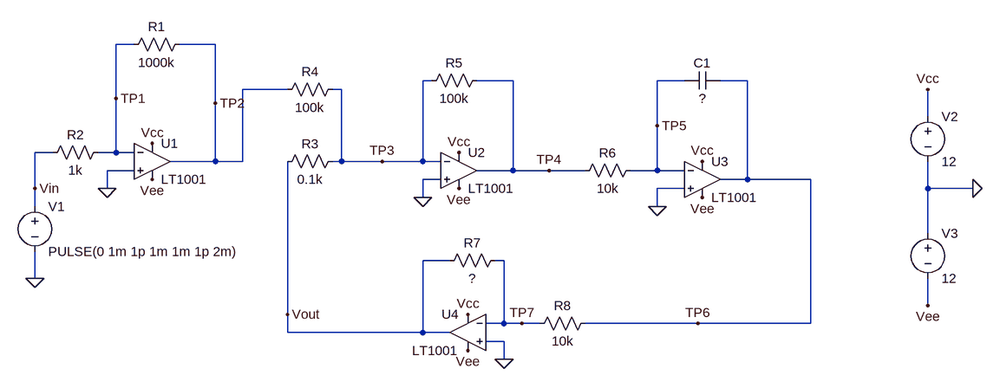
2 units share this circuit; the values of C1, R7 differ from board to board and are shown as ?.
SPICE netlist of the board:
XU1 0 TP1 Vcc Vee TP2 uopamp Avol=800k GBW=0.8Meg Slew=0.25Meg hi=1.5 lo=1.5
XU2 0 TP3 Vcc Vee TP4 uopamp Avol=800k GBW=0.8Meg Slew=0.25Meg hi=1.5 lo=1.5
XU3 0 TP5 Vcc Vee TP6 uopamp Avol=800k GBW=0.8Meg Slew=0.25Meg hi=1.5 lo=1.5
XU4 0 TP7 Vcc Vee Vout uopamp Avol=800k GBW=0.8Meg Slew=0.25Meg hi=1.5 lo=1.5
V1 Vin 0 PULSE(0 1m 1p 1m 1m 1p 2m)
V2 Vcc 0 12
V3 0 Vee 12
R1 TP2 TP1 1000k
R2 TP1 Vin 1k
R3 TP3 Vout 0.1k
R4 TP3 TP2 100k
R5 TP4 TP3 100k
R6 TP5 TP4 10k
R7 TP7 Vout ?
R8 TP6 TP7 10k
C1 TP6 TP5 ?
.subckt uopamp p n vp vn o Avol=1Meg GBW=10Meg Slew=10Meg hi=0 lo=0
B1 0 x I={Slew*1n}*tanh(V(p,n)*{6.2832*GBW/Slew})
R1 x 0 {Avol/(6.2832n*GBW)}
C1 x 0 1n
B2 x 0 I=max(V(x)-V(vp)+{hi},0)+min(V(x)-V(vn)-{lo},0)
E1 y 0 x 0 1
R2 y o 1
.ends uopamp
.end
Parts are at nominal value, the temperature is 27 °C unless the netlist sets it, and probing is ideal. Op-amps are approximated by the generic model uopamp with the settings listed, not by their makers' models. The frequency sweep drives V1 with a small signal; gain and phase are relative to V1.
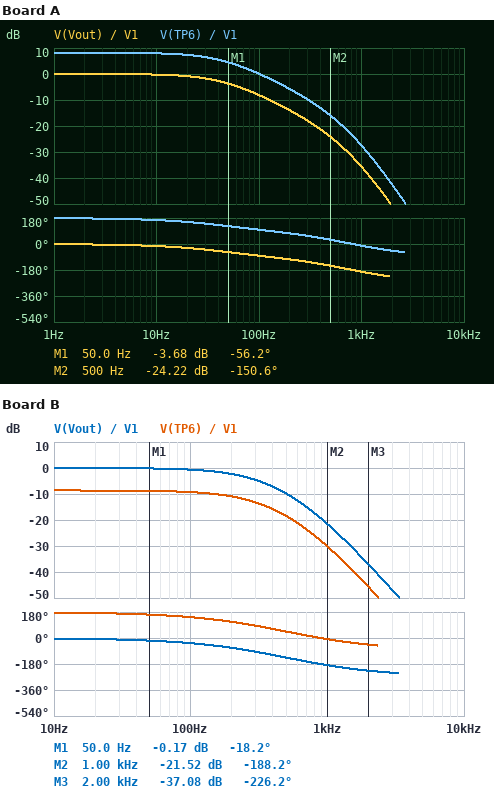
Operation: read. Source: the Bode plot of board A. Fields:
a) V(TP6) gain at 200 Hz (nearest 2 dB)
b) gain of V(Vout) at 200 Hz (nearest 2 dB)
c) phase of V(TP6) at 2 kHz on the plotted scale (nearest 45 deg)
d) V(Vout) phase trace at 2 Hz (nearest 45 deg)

-6 dB
-14 dB
-45 deg
0 deg
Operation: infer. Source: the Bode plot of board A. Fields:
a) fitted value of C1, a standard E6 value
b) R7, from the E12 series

150 µF
3.9 kΩ
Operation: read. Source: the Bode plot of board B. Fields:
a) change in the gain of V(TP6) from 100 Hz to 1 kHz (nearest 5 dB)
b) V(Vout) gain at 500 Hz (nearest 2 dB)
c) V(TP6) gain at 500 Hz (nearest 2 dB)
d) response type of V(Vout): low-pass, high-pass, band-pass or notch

-20 dB
-10 dB
-18 dB
low-pass
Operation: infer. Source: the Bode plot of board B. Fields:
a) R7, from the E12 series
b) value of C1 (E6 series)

27 kΩ
220 µF
